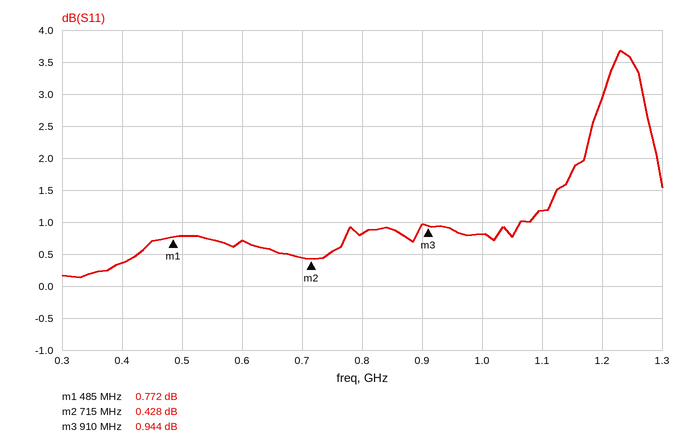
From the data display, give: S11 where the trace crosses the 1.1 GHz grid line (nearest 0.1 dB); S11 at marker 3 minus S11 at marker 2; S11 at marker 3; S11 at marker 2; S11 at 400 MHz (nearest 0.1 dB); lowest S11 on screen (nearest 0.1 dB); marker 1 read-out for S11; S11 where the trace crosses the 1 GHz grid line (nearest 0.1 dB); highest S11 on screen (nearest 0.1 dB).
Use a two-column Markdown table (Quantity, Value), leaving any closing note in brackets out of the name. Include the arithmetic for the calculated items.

| Quantity | Value |
|---|---|
| S11 where the trace crosses the 1.1 GHz grid line | 1.2 dB |
| S11 at marker 3 minus S11 at marker 2 | 0.944 − (0.428) = 0.516 dB |
| S11 at marker 3 | 0.944 dB |
| S11 at marker 2 | 0.428 dB |
| S11 at 400 MHz | 0.4 dB |
| lowest S11 on screen | 0.1 dB |
| marker 1 read-out for S11 | 0.772 dB |
| S11 where the trace crosses the 1 GHz grid line | 0.8 dB |
| highest S11 on screen | 3.7 dB |
